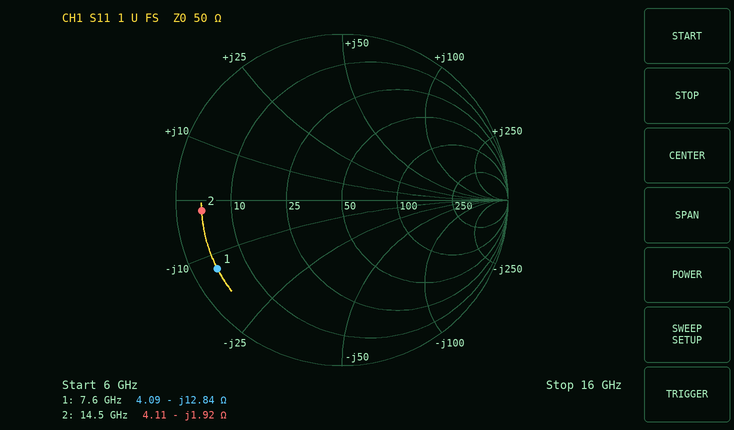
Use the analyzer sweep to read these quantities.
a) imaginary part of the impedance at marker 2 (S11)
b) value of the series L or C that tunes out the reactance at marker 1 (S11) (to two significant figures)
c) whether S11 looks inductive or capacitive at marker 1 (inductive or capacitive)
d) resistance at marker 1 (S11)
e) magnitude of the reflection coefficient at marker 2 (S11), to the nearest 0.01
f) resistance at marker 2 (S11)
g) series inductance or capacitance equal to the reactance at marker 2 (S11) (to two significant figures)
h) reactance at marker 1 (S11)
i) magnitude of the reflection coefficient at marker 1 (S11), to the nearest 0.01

-1.92 Ω
270 pH
capacitive
4.09 Ω
0.85
4.11 Ω
5.7 pF
-12.84 Ω
0.86
